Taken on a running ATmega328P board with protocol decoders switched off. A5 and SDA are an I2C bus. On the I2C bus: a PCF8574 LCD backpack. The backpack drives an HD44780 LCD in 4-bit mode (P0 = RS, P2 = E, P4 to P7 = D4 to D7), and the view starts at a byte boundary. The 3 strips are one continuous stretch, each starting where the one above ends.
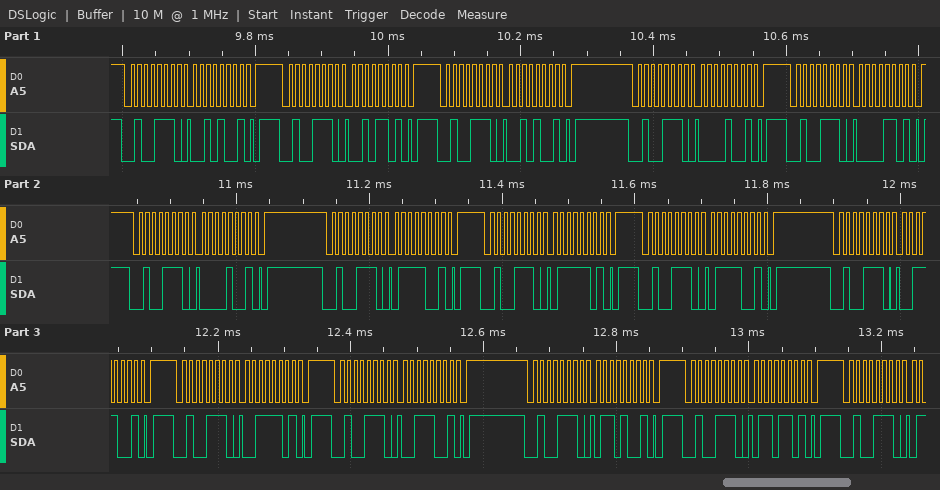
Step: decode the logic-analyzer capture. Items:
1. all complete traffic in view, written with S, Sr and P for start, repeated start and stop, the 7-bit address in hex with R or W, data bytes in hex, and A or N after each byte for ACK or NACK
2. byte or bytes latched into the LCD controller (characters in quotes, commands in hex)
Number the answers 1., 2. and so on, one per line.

1. S 27W A 29 A P S 27W A 2D A P S 27W A 29 A P S 27W A 09 A P S 27W A 0D A P S 27W A 09 A P S 27W A 79 A P S 27W A 7D A P S 27W A 79 A P S 27W A 39 A P S 27W A 3D A P S 27W A 39 A P S 27W A 69 A P S 27W A 6D A P S 27W A
2. ' ' 's'
